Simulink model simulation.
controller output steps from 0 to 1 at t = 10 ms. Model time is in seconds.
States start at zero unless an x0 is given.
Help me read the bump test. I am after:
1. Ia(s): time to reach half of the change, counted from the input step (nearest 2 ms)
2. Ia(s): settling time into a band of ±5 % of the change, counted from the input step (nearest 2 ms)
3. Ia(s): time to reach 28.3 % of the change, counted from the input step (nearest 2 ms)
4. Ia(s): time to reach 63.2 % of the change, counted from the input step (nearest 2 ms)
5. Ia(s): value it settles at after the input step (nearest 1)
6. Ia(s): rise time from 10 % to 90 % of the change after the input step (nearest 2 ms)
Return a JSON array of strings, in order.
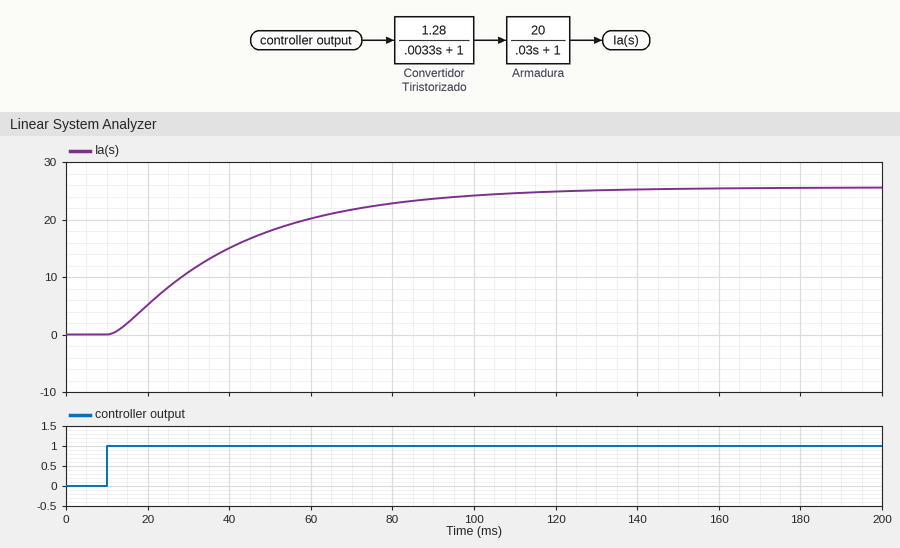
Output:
["24 ms", "94 ms", "14 ms", "34 ms", "26", "66 ms"]
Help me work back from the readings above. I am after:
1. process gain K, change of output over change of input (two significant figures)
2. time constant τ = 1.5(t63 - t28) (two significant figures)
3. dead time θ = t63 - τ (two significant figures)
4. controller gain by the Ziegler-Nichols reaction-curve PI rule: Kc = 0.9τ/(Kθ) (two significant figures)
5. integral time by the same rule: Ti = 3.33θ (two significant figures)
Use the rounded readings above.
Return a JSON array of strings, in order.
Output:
["26", "30 ms", "4.0 ms", "0.26", "13 ms"]
